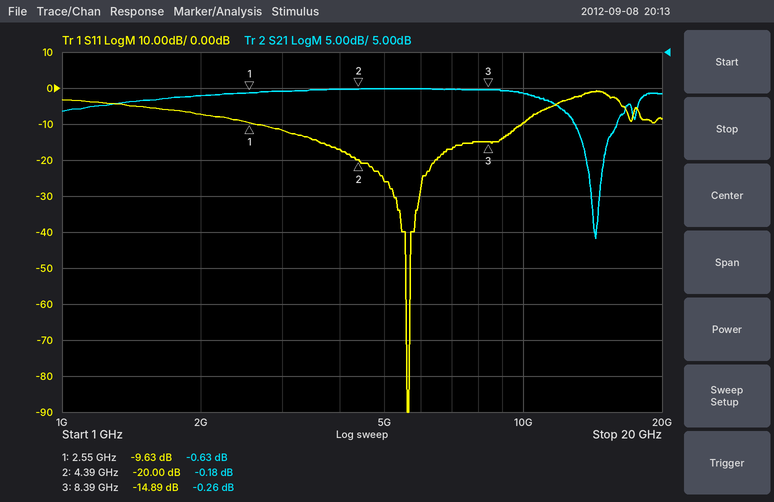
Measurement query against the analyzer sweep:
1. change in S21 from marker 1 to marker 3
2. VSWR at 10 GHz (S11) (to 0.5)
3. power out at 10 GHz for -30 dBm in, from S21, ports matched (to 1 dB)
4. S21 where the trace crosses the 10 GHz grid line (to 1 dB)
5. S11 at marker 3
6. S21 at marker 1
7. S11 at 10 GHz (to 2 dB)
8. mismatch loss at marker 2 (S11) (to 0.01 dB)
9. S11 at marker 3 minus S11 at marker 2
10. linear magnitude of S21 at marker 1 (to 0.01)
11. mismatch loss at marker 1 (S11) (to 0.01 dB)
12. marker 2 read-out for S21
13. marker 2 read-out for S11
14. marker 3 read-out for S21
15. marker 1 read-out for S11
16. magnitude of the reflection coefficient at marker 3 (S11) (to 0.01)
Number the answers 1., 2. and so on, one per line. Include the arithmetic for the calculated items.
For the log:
1. -0.26 − (-0.63) = 0.37 dB
2. |Γ| = 10^(-10/20) = 0.3162; VSWR = (1 + 0.3162)/(1 − 0.3162) ≈ 1.92, so 2.0 to the nearest 0.5
3. -30 dBm + (-1 dB) = -31 dBm
4. -1 dB
5. -14.89 dB
6. -0.63 dB
7. -10 dB
8. −10 log10(1 − 10^(-20/10)) ≈ 0.04 dB
9. -14.89 − (-20) = 5.11 dB
10. 10^(-0.63/20) ≈ 0.93
11. −10 log10(1 − 10^(-9.63/10)) ≈ 0.50 dB
12. -0.18 dB
13. -20.00 dB
14. -0.26 dB
15. -9.63 dB
16. 10^(-14.89/20) ≈ 0.18
